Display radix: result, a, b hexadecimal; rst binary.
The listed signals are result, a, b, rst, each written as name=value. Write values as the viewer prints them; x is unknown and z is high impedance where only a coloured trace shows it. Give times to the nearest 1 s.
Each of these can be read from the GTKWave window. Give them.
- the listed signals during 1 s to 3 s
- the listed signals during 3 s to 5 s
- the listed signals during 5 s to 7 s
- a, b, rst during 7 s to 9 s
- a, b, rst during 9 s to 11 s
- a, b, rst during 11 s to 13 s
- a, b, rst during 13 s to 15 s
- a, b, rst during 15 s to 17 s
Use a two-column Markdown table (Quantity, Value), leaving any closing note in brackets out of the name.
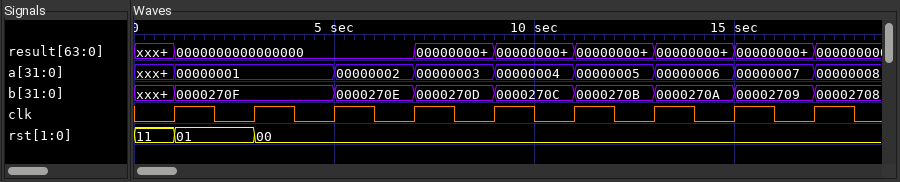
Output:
| Quantity | Value |
|---|---|
| the listed signals during 1 s to 3 s | result=0000000000000000, a=00000001, b=0000270F, rst=01 |
| the listed signals during 3 s to 5 s | result=0000000000000000, a=00000001, b=0000270F, rst=00 |
| the listed signals during 5 s to 7 s | result=0000000000000000, a=00000002, b=0000270E, rst=00 |
| a, b, rst during 7 s to 9 s | a=00000003, b=0000270D, rst=00 |
| a, b, rst during 9 s to 11 s | a=00000004, b=0000270C, rst=00 |
| a, b, rst during 11 s to 13 s | a=00000005, b=0000270B, rst=00 |
| a, b, rst during 13 s to 15 s | a=00000006, b=0000270A, rst=00 |
| a, b, rst during 15 s to 17 s | a=00000007, b=00002709, rst=00 |
